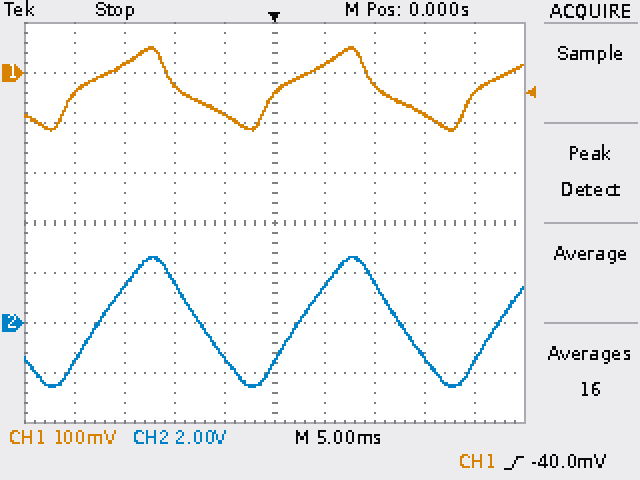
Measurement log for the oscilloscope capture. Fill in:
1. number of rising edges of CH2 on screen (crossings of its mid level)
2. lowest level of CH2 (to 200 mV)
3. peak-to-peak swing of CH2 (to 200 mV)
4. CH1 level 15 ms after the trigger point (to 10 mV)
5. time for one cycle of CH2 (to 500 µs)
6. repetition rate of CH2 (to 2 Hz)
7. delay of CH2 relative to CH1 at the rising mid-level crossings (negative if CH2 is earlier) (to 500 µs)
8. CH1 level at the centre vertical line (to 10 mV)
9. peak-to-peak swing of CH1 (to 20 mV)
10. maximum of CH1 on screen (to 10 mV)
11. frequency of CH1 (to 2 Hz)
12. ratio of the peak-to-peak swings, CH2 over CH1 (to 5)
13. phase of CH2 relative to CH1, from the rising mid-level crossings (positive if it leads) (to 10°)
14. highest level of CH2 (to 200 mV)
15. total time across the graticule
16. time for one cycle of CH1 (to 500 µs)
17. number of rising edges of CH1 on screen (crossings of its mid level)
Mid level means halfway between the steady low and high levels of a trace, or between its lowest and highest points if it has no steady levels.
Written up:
3
-2.6 V
5.2 V
-80 mV
20.0 ms
50 Hz
+2.0 ms
-40 mV
160 mV
50 mV
50 Hz
30
-40°
2.6 V
50 ms
20.0 ms
3
